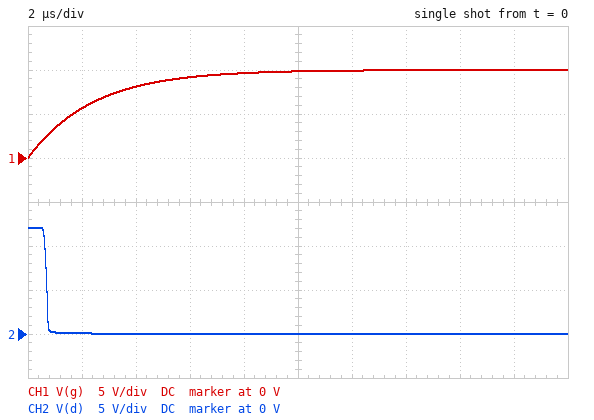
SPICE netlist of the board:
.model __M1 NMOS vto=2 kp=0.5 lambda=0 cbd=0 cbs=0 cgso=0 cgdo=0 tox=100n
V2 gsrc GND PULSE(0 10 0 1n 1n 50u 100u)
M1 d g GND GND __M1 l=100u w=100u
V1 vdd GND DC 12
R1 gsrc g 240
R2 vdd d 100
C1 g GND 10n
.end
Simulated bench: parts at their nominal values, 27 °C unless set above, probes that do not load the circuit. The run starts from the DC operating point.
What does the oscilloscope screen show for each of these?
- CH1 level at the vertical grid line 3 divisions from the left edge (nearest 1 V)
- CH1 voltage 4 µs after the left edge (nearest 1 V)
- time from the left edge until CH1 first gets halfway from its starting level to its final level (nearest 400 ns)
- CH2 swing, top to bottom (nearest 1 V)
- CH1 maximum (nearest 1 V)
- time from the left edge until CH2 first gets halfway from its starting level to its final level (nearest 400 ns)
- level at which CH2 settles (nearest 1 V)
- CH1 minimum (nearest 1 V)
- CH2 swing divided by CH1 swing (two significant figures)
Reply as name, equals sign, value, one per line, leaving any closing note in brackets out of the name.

CH1 level at the vertical grid line 3 divisions from the left edge = 9 V
CH1 voltage 4 µs after the left edge = 8 V
time from the left edge until CH1 first gets halfway from its starting level to its final level = 1.6 µs
CH2 swing, top to bottom = 12 V
CH1 maximum = 10 V
time from the left edge until CH2 first gets halfway from its starting level to its final level = 800 ns
level at which CH2 settles = 0 V
CH1 minimum = 0 V
CH2 swing divided by CH1 swing = 1.2
